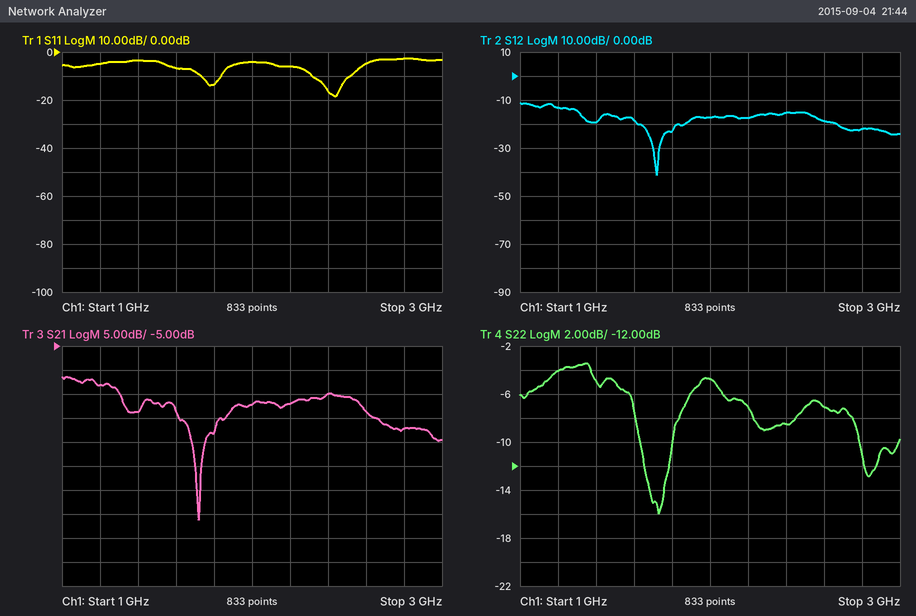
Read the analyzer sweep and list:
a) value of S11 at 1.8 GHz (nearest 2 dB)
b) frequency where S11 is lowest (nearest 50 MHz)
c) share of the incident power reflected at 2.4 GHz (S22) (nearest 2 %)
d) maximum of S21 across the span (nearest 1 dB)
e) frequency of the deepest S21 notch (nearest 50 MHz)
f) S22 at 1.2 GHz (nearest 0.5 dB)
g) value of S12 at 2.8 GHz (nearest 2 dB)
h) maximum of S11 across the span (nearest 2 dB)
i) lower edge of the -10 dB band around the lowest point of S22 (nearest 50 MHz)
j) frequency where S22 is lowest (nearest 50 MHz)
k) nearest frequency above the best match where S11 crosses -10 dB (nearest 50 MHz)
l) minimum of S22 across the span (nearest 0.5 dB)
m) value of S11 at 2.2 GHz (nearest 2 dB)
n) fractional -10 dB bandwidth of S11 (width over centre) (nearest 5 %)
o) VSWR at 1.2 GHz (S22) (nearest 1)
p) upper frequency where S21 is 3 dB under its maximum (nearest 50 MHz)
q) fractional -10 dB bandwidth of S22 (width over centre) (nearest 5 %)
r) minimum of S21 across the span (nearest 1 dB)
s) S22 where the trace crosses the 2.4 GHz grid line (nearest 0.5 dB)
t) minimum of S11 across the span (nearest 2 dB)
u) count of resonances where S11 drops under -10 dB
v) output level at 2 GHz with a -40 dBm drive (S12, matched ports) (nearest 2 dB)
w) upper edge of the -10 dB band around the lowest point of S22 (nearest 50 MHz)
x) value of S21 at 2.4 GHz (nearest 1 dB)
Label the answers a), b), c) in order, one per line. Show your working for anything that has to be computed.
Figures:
a) -14 dB
b) 2.45 GHz
c) 10^(-8.5/10) ≈ 14 %
d) -11 dB
e) 1.70 GHz
f) -4.0 dB
g) -22 dB
h) -2 dB
i) 1.65 GHz
j) 1.75 GHz
k) 2.50 GHz
l) -16.0 dB
m) -6 dB
n) 200 MHz / 2.4 GHz ≈ 8.33 %, so 10 % to the nearest 5 %
o) |Γ| = 10^(-4/20) = 0.6310; VSWR = (1 + 0.6310)/(1 − 0.6310) ≈ 4
p) 1.30 GHz
q) 150 MHz / 1.725 GHz ≈ 8.70 %, so 10 % to the nearest 5 %
r) -41 dB
s) -8.5 dB
t) -18 dB
u) 2
v) -40 dBm + (-18 dB) = -58 dBm
w) 1.80 GHz
x) -15 dB
